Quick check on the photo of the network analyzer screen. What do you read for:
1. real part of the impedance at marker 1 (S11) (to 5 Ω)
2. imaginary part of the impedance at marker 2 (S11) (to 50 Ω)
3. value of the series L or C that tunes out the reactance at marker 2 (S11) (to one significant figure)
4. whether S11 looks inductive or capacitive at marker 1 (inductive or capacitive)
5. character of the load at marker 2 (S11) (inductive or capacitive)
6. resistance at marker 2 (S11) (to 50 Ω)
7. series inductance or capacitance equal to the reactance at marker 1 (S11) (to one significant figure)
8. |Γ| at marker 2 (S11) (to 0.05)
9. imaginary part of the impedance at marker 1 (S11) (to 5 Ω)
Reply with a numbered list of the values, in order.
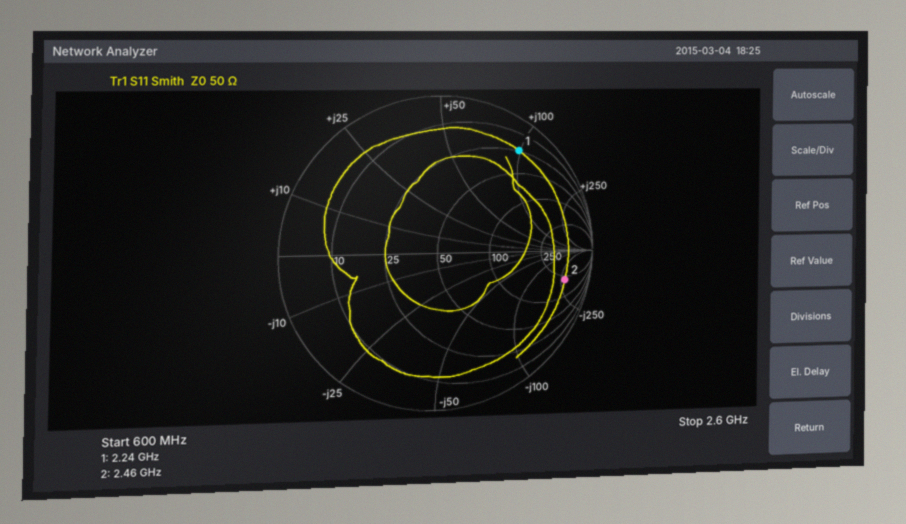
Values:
1. 25 Ω
2. -300 Ω
3. 20 nH
4. inductive
5. capacitive
6. 200 Ω
7. 7 nH
8. 0.85
9. +100 Ω
